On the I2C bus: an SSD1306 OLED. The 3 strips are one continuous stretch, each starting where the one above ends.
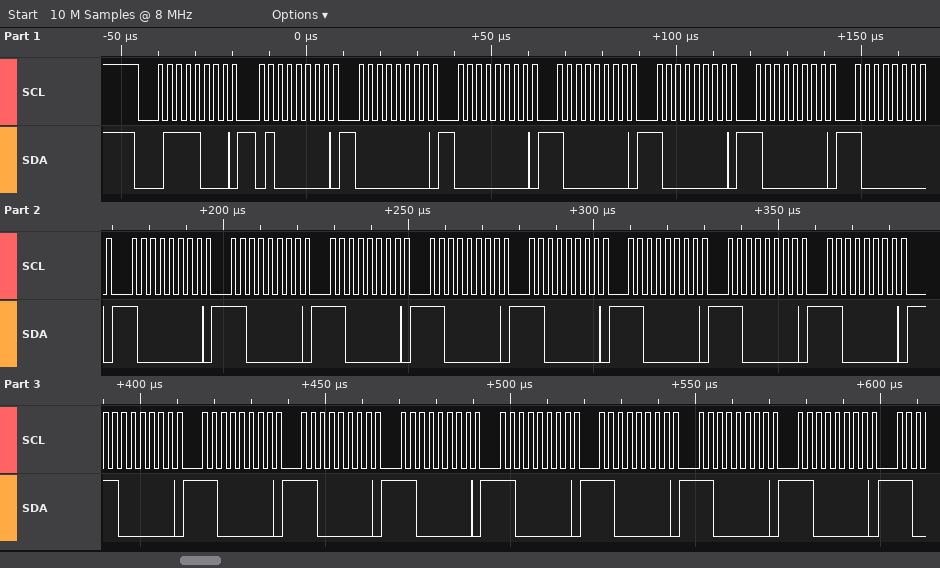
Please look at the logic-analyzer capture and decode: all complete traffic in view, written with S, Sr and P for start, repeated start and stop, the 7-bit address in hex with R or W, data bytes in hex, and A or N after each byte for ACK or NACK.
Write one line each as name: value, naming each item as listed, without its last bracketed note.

all complete traffic in view, written with S, Sr and P for start, repeated start and stop, the 7-bit address in hex with R or W, data bytes in hex, and A or N after each byte for ACK or NACK: S 3CW A 40 A 00 A 00 A 80 A 80 A 80 A 80 A 80 A C0 A C0 A C0 A C0 A C0 A C0 A C0 A C0 A C0 A C0 A C0 A C0 A C0 A C0 A C0 A
